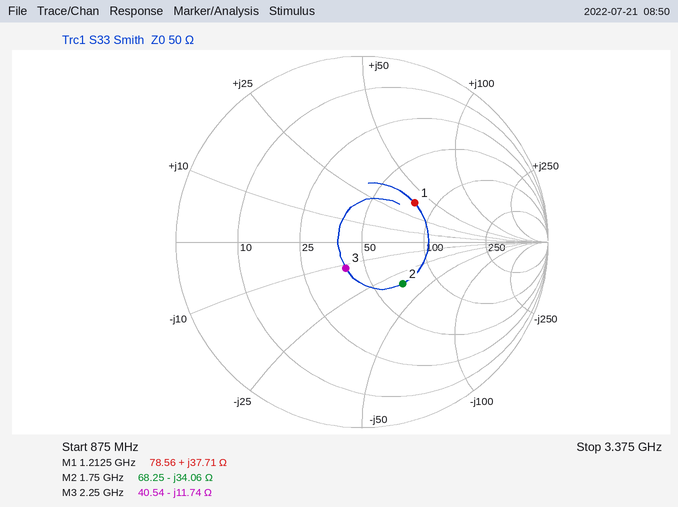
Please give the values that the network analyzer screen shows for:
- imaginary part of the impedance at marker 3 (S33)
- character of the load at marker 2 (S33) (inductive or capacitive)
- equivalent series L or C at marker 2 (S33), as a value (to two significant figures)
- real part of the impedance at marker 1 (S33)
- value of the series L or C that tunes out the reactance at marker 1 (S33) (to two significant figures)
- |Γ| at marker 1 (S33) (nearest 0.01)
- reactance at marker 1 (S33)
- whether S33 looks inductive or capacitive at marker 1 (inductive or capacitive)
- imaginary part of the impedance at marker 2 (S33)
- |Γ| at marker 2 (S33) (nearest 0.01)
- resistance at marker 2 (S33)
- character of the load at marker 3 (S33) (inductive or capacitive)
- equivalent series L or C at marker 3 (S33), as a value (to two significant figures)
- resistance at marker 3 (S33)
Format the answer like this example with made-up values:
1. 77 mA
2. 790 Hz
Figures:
1. -11.74 Ω
2. capacitive
3. 2.7 pF
4. 78.56 Ω
5. 3.5 pF
6. 0.35
7. +37.71 Ω
8. inductive
9. -34.06 Ω
10. 0.31
11. 68.25 Ω
12. capacitive
13. 6.0 pF
14. 40.54 Ω
